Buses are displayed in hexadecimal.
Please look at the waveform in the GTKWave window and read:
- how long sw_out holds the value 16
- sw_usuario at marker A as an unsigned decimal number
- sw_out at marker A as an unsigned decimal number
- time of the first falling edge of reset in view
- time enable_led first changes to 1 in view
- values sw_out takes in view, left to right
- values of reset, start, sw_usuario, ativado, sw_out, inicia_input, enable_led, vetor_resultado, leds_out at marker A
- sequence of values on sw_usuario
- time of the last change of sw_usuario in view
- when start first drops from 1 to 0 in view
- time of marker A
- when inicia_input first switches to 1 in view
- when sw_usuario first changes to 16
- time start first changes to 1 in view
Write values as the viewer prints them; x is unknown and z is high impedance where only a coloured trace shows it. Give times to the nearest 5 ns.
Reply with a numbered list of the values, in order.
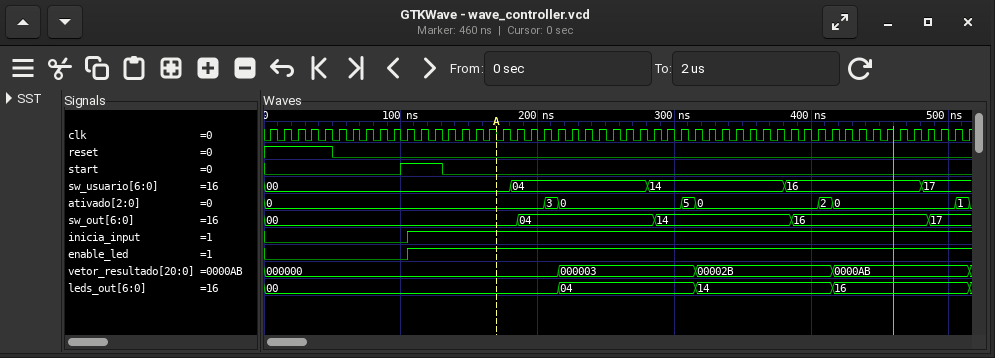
1. 100 ns
2. 0
3. 0
4. 50 ns
5. 105 ns
6. 00, 04, 14, 16, 17
7. reset=0, start=0, sw_usuario=00, ativado=0, sw_out=00, inicia_input=1, enable_led=1, vetor_resultado=000000, leds_out=00
8. 00, 04, 14, 16, 17
9. 480 ns
10. 130 ns
11. 170 ns
12. 105 ns
13. 380 ns
14. 100 ns
